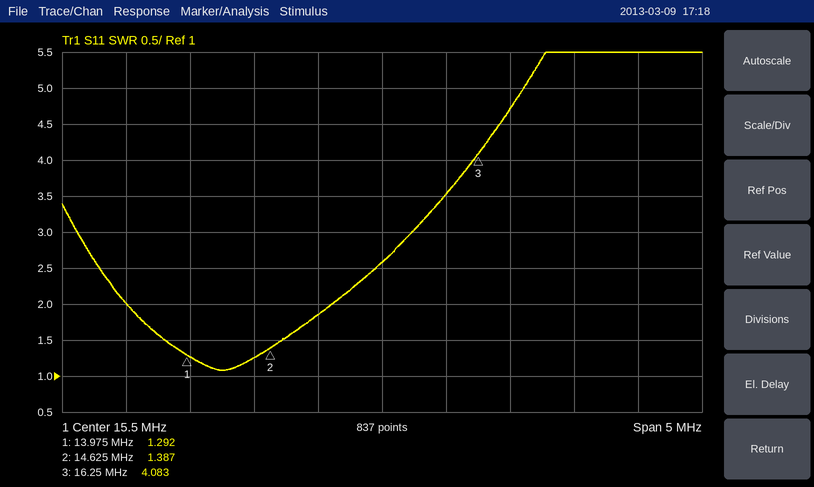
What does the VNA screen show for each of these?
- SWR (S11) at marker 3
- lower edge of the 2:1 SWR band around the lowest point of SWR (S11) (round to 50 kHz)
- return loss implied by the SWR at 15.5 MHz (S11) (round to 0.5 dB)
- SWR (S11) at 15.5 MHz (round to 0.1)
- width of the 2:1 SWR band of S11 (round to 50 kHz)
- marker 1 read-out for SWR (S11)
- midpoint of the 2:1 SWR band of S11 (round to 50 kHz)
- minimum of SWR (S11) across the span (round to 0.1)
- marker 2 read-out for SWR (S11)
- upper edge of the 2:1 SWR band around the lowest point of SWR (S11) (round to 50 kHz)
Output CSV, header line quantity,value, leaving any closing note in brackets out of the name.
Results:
quantity,value
SWR (S11) at marker 3,4.083
lower edge of the 2:1 SWR band around the lowest point of SWR (S11),13.50 MHz
return loss implied by the SWR at 15.5 MHz (S11),7.0 dB
SWR (S11) at 15.5 MHz,2.6
width of the 2:1 SWR band of S11,1.60 MHz
marker 1 read-out for SWR,1.292
midpoint of the 2:1 SWR band of S11,14.30 MHz
minimum of SWR (S11) across the span,1.1
marker 2 read-out for SWR,1.387
upper edge of the 2:1 SWR band around the lowest point of SWR (S11),15.10 MHz
